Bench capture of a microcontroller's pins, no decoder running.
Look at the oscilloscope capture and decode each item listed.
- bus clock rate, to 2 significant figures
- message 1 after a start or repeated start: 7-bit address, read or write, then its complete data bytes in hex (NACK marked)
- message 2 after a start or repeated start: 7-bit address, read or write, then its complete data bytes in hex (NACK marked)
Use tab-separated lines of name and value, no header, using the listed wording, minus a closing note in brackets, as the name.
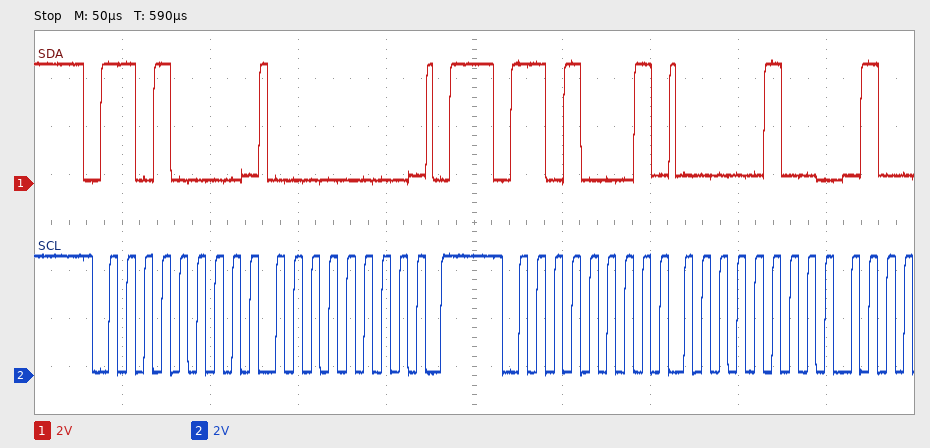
bus clock rate, to 2 significant figures	100 kHz
message 1 after a start or repeated start: 7-bit address, read or write, then its complete data bytes in hex	0x68 write: 00
message 2 after a start or repeated start: 7-bit address, read or write, then its complete data bytes in hex	0x68 read: 04
